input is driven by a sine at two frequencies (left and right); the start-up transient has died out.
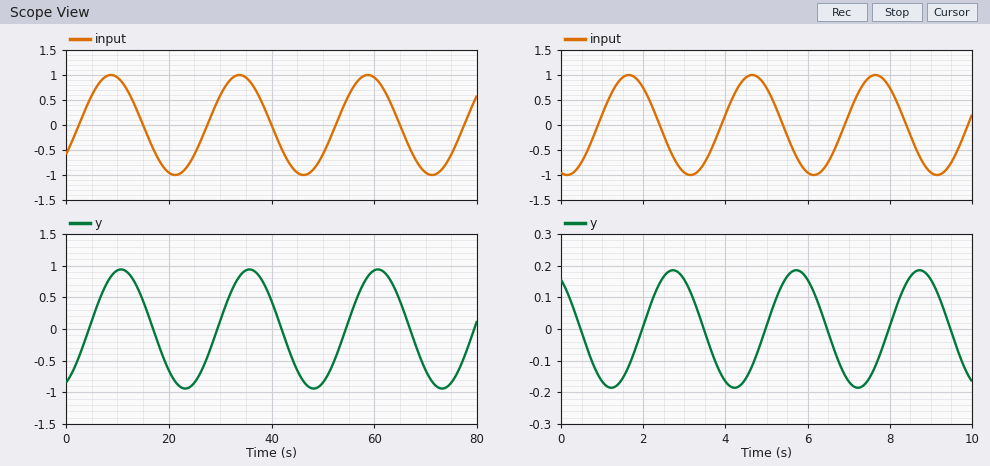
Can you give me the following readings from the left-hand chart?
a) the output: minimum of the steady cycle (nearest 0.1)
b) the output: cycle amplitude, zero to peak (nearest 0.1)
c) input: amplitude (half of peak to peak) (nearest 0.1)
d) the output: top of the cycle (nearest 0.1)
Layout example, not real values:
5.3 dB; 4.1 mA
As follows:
-0.9; 0.9; 1.0; 0.9
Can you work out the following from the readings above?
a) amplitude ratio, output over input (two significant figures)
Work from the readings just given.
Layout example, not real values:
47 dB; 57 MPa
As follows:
0.90
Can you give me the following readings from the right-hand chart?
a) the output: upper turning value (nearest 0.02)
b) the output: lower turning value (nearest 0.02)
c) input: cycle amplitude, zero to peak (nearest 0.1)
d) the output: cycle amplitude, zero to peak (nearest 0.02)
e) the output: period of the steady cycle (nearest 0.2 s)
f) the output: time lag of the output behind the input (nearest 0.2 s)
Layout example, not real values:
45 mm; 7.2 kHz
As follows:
0.18; -0.18; 1.0; 0.18; 3.0 s; 1.0 s
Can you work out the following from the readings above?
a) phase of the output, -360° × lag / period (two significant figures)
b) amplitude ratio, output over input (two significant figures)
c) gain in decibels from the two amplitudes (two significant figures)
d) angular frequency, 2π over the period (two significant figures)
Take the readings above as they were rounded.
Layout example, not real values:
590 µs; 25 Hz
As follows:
-120°; 0.18; -15 dB; 2.1 rad/s
